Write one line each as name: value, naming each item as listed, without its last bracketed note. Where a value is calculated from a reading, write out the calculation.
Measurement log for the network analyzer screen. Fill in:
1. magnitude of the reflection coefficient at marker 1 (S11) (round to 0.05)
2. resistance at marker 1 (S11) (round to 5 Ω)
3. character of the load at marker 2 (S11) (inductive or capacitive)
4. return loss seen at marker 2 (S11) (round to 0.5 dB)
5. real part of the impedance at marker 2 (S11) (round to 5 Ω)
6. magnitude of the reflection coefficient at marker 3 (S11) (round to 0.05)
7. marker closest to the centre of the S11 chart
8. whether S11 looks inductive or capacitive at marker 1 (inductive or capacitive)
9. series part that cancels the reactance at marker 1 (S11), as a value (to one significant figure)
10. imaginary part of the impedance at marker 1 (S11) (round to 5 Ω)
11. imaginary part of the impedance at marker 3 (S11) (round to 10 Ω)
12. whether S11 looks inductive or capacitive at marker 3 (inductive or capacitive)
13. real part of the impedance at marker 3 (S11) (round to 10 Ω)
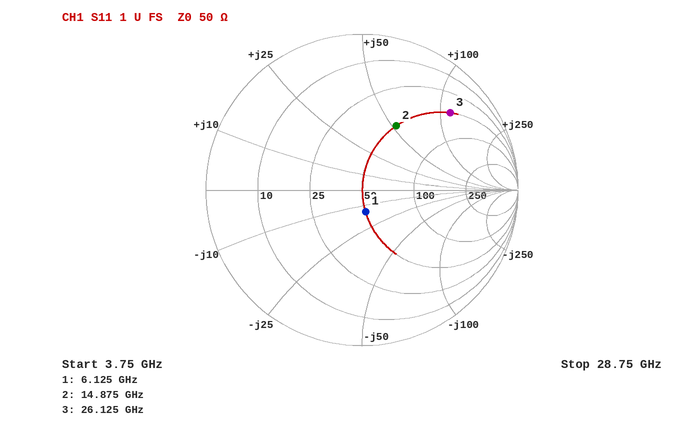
magnitude of the reflection coefficient at marker 1 (S11): 0.15
resistance at marker 1 (S11): 50 Ω
character of the load at marker 2 (S11): inductive
return loss seen at marker 2 (S11): 6.5 dB
real part of the impedance at marker 2 (S11): 50 Ω
magnitude of the reflection coefficient at marker 3 (S11): 0.75
marker closest to the centre of the S11 chart: marker 1
whether S11 looks inductive or capacitive at marker 1: capacitive
series part that cancels the reactance at marker 1 (S11), as a value: L = 15 Ω/(2π × 6.125 GHz) ≈ 390 pH, so 400 pH to one significant figure
imaginary part of the impedance at marker 1 (S11): -15 Ω
imaginary part of the impedance at marker 3 (S11): +110 Ω
whether S11 looks inductive or capacitive at marker 3: inductive
real part of the impedance at marker 3 (S11): 50 Ω
